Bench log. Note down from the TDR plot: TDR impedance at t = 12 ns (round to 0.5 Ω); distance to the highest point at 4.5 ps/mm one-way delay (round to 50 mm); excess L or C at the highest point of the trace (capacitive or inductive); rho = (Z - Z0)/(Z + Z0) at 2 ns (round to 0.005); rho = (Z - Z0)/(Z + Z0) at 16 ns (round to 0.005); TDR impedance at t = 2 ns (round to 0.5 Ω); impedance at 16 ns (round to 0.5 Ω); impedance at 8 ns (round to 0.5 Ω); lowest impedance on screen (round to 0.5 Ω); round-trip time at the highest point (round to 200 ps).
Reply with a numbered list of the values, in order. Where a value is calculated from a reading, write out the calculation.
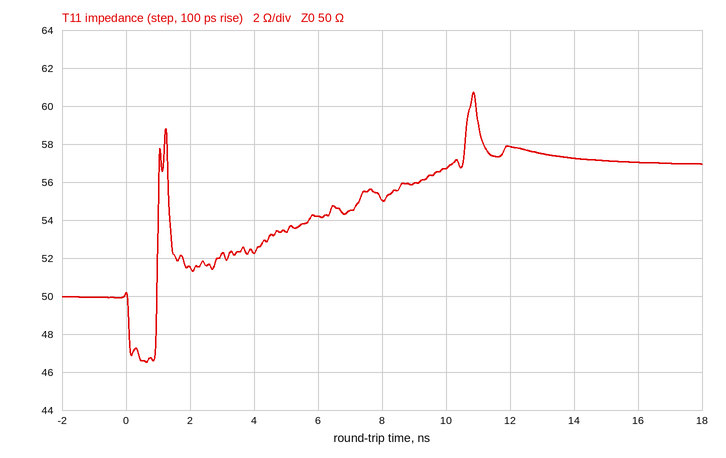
1. 58.0 Ω
2. 10.8 ns / 2 / 4.5 ps/mm ≈ 1.20 m
3. inductive
4. (51.5 − 50)/(51.5 + 50) ≈ +0.015
5. (57 − 50)/(57 + 50) ≈ +0.065
6. 51.5 Ω
7. 57.0 Ω
8. 55.0 Ω
9. 46.5 Ω
10. 10.8 ns
